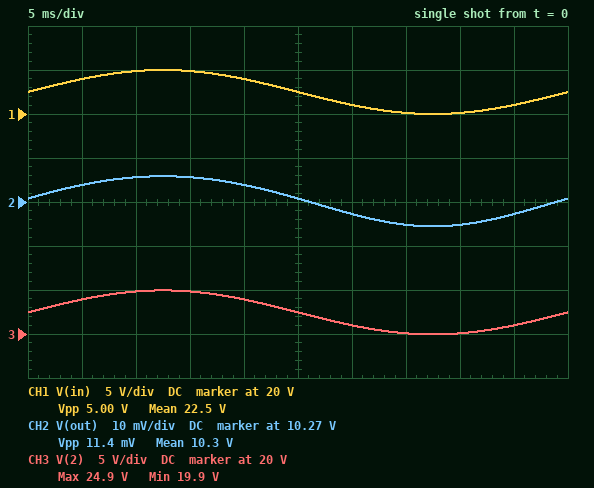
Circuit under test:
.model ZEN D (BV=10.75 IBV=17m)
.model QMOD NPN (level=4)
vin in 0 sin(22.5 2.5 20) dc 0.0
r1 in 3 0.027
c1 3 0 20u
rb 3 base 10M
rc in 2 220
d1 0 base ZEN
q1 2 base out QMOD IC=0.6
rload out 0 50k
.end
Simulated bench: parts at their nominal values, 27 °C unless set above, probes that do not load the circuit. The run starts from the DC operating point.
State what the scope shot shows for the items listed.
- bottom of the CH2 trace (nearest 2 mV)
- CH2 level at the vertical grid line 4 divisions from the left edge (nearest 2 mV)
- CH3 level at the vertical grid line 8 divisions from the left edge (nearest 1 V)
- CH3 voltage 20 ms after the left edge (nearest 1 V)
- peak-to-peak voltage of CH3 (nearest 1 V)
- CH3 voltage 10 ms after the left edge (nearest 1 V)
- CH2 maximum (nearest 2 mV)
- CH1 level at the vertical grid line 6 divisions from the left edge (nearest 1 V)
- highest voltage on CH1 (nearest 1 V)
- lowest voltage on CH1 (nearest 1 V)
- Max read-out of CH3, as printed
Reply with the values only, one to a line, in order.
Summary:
10.264 V
10.274 V
20 V
24 V
5 V
25 V
10.276 V
21 V
25 V
20 V
24.9 V
